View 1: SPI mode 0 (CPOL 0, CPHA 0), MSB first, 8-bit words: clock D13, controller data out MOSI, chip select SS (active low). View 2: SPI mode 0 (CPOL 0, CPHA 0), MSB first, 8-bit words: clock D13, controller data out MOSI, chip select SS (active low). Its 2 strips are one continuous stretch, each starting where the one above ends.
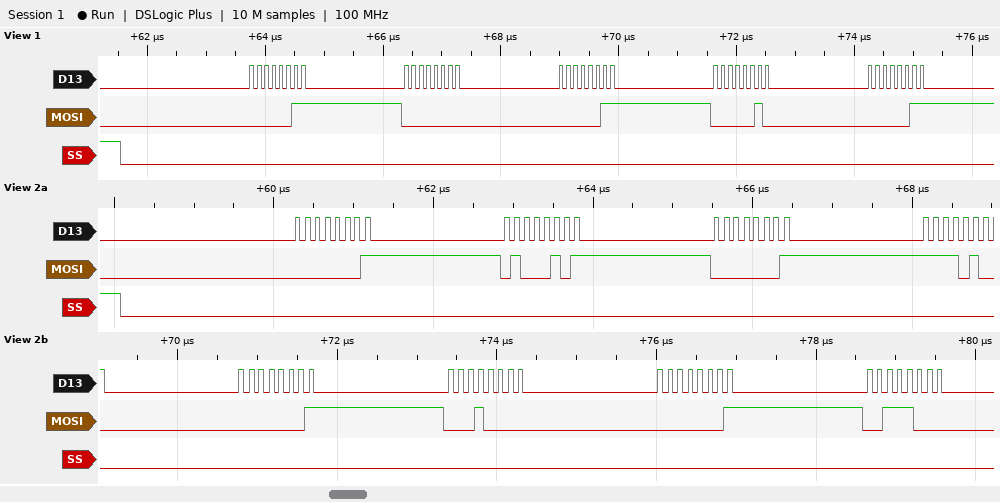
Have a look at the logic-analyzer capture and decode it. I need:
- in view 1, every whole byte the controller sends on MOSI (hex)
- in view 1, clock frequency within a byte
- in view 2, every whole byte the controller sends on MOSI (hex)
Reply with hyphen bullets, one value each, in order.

- 03 00 03 02 03
- 8 MHz
- 01 45 01 F4 01 10 01 38
